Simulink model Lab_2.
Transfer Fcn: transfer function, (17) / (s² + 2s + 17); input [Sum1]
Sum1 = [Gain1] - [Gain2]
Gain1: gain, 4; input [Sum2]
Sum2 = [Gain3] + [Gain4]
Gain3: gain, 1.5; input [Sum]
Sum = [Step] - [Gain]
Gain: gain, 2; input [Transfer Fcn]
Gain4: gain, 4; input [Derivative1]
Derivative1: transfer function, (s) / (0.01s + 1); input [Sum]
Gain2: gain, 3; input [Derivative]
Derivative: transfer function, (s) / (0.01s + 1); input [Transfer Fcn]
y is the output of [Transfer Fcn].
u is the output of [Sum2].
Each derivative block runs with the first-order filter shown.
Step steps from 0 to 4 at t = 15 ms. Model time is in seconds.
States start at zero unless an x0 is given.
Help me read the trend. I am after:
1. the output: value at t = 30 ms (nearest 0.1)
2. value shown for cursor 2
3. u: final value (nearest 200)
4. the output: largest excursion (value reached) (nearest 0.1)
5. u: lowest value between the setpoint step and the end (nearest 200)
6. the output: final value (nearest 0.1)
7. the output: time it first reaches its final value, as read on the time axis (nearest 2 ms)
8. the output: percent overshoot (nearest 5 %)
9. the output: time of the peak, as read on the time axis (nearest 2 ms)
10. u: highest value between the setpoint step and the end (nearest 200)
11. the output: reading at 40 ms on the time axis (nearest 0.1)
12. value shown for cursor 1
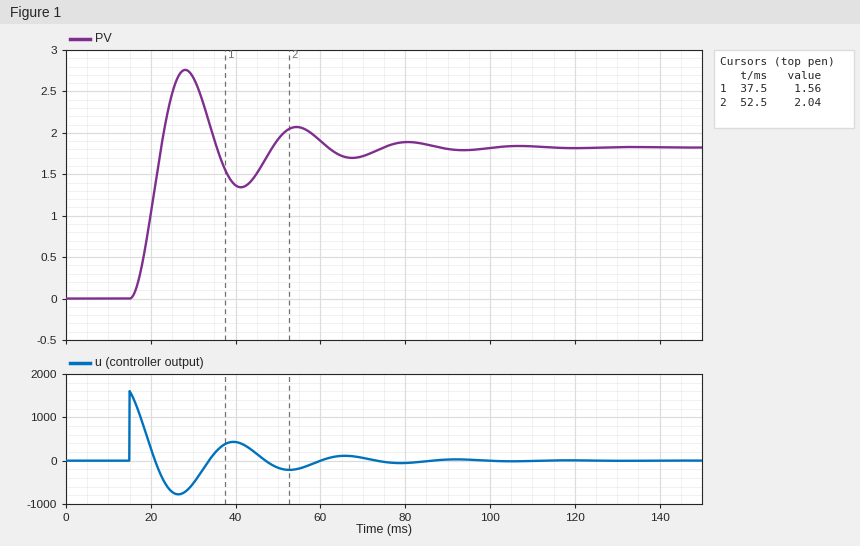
2.7
2.04
0
2.8
-800
1.8
22 ms
50 %
28 ms
1600
1.4
1.56
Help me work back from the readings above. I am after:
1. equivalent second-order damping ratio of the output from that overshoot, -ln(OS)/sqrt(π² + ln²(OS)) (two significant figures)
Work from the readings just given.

0.22
